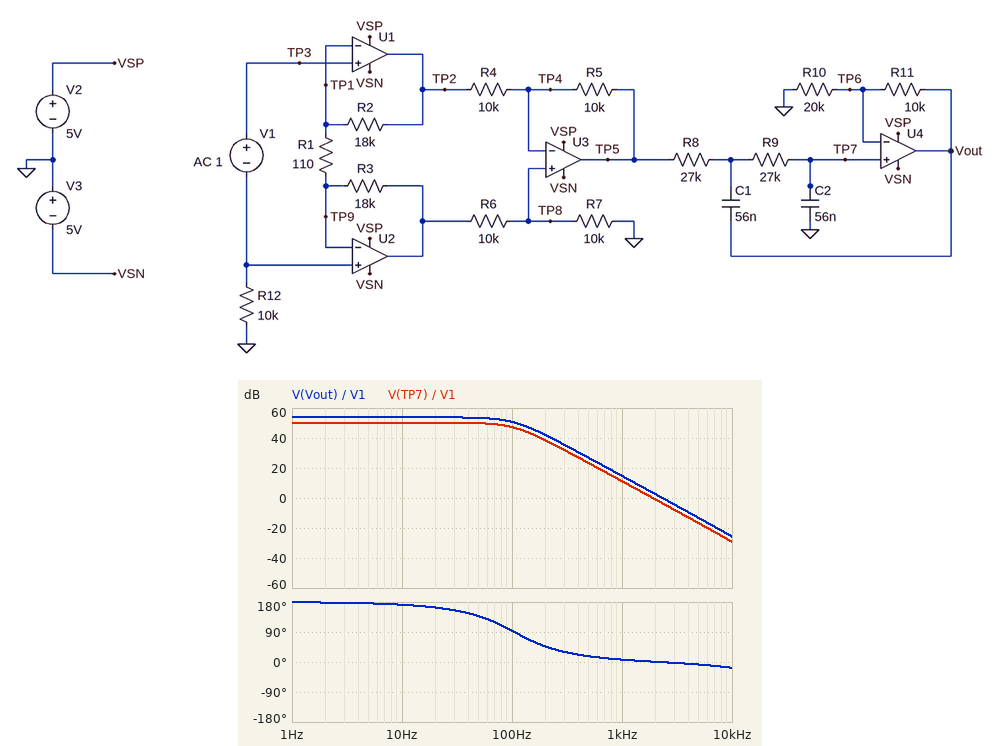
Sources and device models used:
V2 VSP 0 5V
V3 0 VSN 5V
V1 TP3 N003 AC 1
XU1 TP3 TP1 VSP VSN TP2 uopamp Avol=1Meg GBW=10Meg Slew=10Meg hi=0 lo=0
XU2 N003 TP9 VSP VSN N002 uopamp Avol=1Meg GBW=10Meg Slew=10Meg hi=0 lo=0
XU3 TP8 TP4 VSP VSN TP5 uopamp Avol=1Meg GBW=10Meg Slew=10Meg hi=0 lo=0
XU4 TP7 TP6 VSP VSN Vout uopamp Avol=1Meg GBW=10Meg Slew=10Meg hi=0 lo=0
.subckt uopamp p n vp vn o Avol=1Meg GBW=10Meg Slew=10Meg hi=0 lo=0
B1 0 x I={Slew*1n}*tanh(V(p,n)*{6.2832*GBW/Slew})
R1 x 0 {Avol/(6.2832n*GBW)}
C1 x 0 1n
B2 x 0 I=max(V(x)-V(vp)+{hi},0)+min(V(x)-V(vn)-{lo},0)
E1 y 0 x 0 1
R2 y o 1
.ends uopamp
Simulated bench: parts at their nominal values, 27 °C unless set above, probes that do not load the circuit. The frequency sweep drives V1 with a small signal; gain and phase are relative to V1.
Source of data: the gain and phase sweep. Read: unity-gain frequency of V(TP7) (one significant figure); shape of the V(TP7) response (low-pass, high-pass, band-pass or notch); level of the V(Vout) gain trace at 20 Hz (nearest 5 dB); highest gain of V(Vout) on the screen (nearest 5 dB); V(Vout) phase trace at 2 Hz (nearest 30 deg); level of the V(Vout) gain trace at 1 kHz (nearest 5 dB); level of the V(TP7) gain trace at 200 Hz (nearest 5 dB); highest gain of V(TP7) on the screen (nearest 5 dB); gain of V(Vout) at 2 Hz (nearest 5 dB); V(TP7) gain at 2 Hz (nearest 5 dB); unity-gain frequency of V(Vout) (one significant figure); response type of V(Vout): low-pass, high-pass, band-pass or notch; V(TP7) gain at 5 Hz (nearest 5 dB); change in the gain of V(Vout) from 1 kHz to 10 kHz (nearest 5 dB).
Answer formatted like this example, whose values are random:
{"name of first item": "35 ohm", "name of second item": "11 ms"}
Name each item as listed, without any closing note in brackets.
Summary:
{"unity-gain frequency of V(TP7)": "2 kHz", "shape of the V(TP7) response": "low-pass", "level of the V(Vout) gain trace at 20 Hz": "55 dB", "highest gain of V(Vout) on the screen": "55 dB", "V(Vout) phase trace at 2 Hz": "180 deg", "level of the V(Vout) gain trace at 1 kHz": "15 dB", "level of the V(TP7) gain trace at 200 Hz": "40 dB", "highest gain of V(TP7) on the screen": "50 dB", "gain of V(Vout) at 2 Hz": "55 dB", "V(TP7) gain at 2 Hz": "50 dB", "unity-gain frequency of V(Vout)": "2 kHz", "response type of V(Vout): low-pass, high-pass, band-pass or notch": "low-pass", "V(TP7) gain at 5 Hz": "50 dB", "change in the gain of V(Vout) from 1 kHz to 10 kHz": "-40 dB"}
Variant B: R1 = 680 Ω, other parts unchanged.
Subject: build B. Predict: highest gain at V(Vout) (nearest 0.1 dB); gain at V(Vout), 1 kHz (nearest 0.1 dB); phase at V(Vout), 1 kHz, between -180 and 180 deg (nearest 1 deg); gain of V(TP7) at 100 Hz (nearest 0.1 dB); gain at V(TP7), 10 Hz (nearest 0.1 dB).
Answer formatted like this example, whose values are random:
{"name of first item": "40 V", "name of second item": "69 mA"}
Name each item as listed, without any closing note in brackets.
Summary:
{"highest gain at V(Vout)": "38.2 dB", "gain at V(Vout), 1 kHz": "-1.0 dB", "phase at V(Vout), 1 kHz, between -180 and 180 deg": "9 deg", "gain of V(TP7) at 100 Hz": "31.5 dB", "gain at V(TP7), 10 Hz": "34.6 dB"}
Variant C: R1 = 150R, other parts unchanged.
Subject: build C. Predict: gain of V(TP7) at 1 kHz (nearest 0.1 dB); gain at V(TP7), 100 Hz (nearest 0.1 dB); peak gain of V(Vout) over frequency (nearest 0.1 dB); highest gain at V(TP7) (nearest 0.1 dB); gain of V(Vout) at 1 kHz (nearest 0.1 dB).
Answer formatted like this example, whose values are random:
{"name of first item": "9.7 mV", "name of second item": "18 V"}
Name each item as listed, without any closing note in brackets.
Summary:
{"gain of V(TP7) at 1 kHz": "8.5 dB", "gain at V(TP7), 100 Hz": "44.5 dB", "peak gain of V(Vout) over frequency": "51.2 dB", "highest gain at V(TP7)": "47.6 dB", "gain of V(Vout) at 1 kHz": "12.0 dB"}
